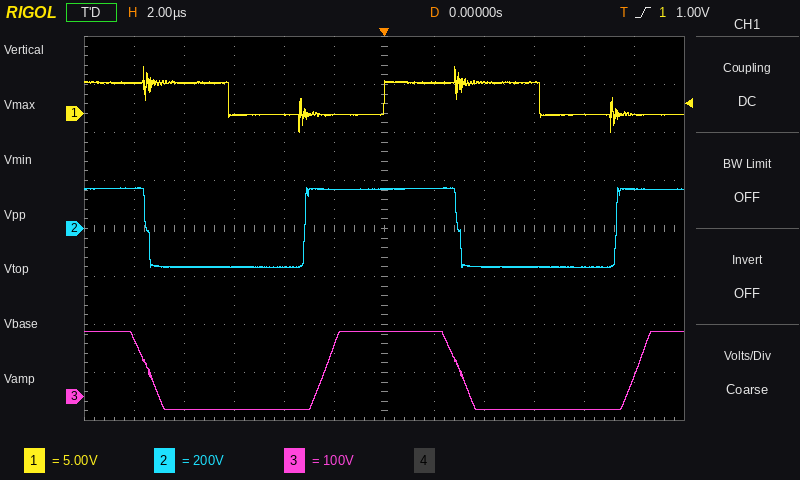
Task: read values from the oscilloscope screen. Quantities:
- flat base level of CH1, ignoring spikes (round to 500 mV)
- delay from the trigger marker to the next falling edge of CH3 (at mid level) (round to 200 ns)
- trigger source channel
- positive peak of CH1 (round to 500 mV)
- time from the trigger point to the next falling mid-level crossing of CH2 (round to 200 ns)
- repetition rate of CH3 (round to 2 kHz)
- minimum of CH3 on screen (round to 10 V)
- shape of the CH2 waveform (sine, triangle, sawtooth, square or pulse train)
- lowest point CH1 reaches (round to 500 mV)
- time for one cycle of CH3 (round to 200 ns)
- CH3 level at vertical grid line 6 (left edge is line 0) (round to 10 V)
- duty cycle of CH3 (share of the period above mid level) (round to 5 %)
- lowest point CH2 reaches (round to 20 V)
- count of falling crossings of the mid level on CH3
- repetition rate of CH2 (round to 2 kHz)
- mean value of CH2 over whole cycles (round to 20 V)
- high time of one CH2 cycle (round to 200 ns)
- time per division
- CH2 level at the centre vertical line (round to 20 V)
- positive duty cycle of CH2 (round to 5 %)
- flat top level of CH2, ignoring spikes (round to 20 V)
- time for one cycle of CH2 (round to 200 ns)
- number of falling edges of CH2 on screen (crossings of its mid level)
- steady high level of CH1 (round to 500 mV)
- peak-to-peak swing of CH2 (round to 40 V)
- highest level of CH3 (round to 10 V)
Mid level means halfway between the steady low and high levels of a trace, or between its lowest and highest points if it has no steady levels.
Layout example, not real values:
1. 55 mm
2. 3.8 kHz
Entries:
1. 0.0 V
2. 3.0 µs
3. CH1
4. 5.0 V
5. 3.0 µs
6. 80 kHz
7. -30 V
8. square
9. -2.0 V
10. 12.4 µs
11. 140 V
12. 45 %
13. -160 V
14. 2
15. 80 kHz
16. 0 V
17. 6.2 µs
18. 2 µs
19. 160 V
20. 50 %
21. 160 V
22. 12.4 µs
23. 2
24. 3.0 V
25. 320 V
26. 140 V
